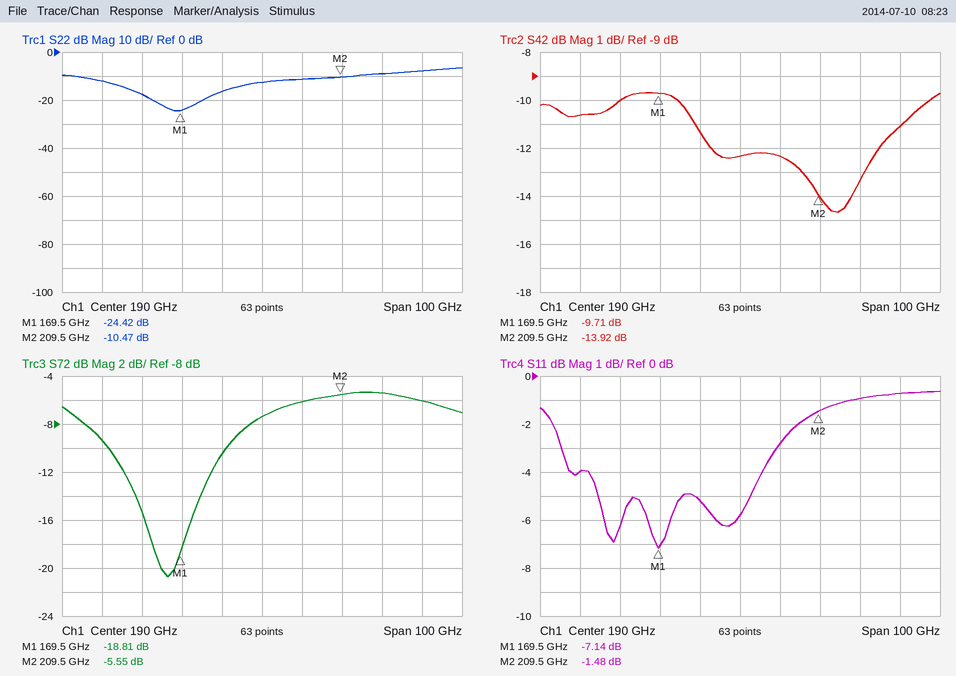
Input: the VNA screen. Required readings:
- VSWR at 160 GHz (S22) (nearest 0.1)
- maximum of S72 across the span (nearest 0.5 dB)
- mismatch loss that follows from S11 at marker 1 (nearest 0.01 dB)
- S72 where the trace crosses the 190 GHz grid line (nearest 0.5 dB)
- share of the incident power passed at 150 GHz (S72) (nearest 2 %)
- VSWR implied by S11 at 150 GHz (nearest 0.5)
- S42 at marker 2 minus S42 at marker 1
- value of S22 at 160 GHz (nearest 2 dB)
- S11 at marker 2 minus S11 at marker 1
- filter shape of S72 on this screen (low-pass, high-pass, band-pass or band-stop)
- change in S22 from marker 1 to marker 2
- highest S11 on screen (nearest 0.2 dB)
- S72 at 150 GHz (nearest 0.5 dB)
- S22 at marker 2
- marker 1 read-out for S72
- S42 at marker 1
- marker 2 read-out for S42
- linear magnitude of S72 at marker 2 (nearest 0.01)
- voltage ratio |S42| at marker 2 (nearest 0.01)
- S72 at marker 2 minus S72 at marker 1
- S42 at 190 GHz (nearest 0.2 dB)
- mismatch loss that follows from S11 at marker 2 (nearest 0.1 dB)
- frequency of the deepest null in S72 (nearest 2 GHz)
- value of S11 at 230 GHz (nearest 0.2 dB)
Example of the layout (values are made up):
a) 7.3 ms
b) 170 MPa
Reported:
a) 1.3
b) -5.5 dB
c) 0.93 dB
d) -7.5 dB
e) 12 %
f) 4.5
g) -4.21 dB
h) -18 dB
i) 5.66 dB
j) band-stop
k) 13.95 dB
l) -0.6 dB
m) -9.5 dB
n) -10.47 dB
o) -18.81 dB
p) -9.71 dB
q) -13.92 dB
r) 0.53
s) 0.20
t) 13.26 dB
u) -12.4 dB
v) 5.4 dB
w) 166 GHz
x) -0.8 dB
